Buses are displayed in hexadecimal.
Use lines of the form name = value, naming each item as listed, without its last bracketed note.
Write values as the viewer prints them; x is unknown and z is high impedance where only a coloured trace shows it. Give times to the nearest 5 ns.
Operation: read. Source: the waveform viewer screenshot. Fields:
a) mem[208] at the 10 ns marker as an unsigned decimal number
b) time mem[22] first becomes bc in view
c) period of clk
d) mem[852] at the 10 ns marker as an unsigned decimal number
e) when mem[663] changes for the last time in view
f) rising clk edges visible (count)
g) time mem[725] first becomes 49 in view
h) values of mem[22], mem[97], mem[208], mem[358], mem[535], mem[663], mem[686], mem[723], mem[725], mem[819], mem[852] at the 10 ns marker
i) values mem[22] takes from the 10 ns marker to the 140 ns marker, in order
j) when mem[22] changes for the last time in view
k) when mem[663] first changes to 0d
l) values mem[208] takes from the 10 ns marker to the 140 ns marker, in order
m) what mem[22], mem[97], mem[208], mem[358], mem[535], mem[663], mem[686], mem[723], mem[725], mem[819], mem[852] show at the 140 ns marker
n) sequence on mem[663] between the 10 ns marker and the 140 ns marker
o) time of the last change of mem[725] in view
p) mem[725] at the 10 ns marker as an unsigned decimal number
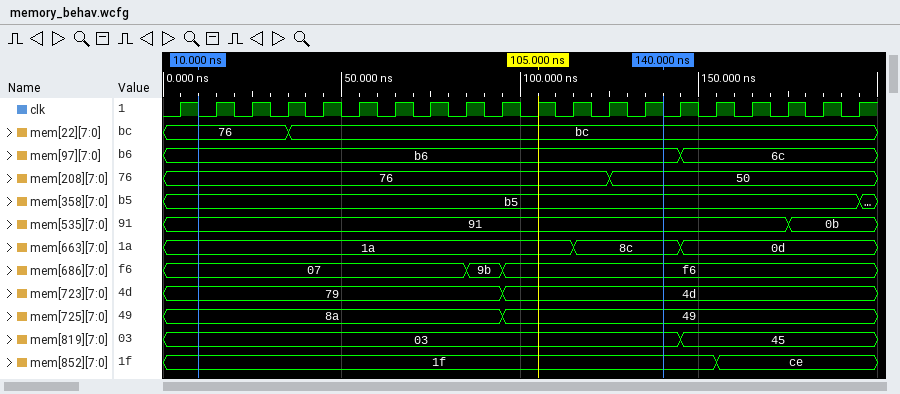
mem[208] at the 10 ns marker as an unsigned decimal number = 118
time mem[22] first becomes bc in view = 35 ns
period of clk = 10 ns
mem[852] at the 10 ns marker as an unsigned decimal number = 31
when mem[663] changes for the last time in view = 145 ns
rising clk edges visible = 20
time mem[725] first becomes 49 in view = 95 ns
values of mem[22], mem[97], mem[208], mem[358], mem[535], mem[663], mem[686], mem[723], mem[725], mem[819], mem[852] at the 10 ns marker = mem[22]=76, mem[97]=b6, mem[208]=76, mem[358]=b5, mem[535]=91, mem[663]=1a, mem[686]=07, mem[723]=79, mem[725]=8a, mem[819]=03, mem[852]=1f
values mem[22] takes from the 10 ns marker to the 140 ns marker, in order = 76, bc
when mem[22] changes for the last time in view = 35 ns
when mem[663] first changes to 0d = 145 ns
values mem[208] takes from the 10 ns marker to the 140 ns marker, in order = 76, 50
what mem[22], mem[97], mem[208], mem[358], mem[535], mem[663], mem[686], mem[723], mem[725], mem[819], mem[852] show at the 140 ns marker = mem[22]=bc, mem[97]=b6, mem[208]=50, mem[358]=b5, mem[535]=91, mem[663]=8c, mem[686]=f6, mem[723]=4d, mem[725]=49, mem[819]=03, mem[852]=1f
sequence on mem[663] between the 10 ns marker and the 140 ns marker = 1a, 8c
time of the last change of mem[725] in view = 95 ns
mem[725] at the 10 ns marker as an unsigned decimal number = 138
